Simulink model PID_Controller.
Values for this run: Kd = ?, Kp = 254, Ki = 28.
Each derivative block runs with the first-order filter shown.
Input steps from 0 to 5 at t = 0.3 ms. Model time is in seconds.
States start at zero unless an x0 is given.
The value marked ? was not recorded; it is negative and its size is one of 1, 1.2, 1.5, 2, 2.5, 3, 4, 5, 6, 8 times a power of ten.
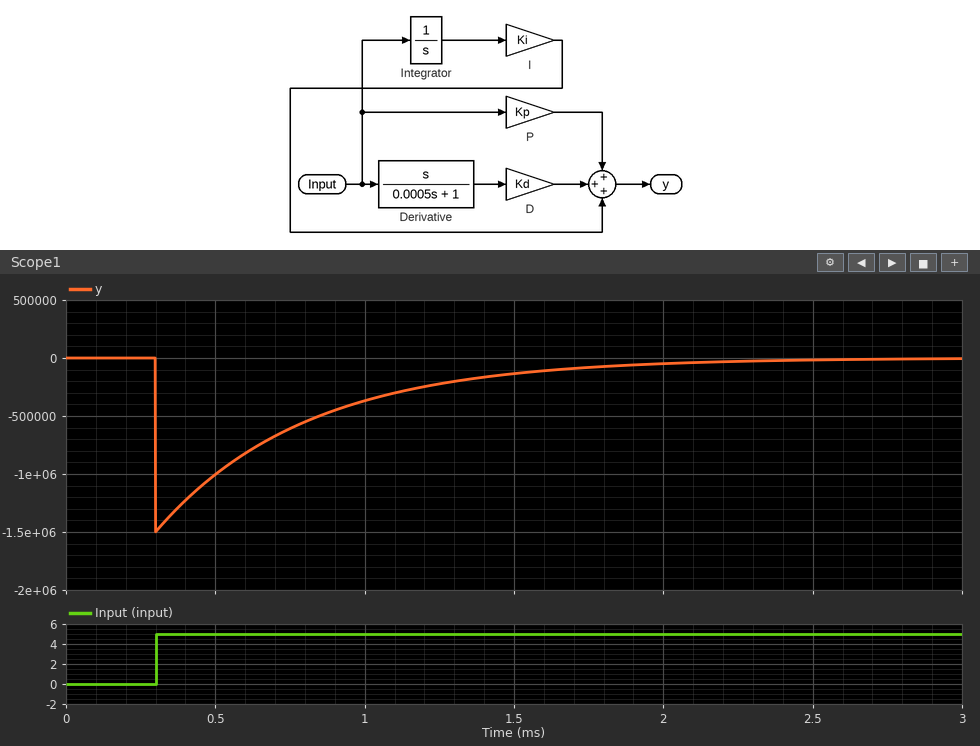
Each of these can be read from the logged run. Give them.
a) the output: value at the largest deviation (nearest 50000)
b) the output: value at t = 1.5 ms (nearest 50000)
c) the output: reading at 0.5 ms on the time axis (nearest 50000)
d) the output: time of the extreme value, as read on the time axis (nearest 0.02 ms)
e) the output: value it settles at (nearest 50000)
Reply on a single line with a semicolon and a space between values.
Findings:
-1500000; -150000; -1000000; 0.30 ms; 0
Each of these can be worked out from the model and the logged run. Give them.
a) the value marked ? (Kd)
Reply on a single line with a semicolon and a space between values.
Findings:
-150
